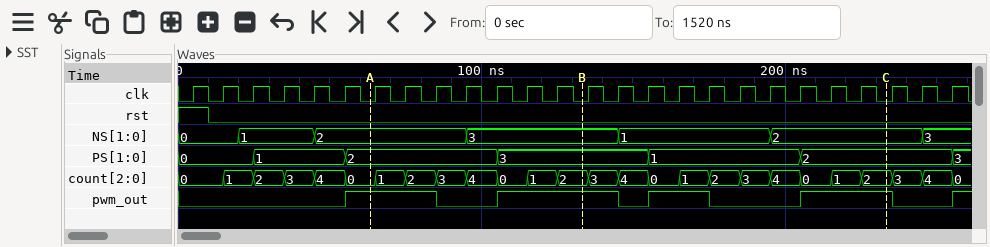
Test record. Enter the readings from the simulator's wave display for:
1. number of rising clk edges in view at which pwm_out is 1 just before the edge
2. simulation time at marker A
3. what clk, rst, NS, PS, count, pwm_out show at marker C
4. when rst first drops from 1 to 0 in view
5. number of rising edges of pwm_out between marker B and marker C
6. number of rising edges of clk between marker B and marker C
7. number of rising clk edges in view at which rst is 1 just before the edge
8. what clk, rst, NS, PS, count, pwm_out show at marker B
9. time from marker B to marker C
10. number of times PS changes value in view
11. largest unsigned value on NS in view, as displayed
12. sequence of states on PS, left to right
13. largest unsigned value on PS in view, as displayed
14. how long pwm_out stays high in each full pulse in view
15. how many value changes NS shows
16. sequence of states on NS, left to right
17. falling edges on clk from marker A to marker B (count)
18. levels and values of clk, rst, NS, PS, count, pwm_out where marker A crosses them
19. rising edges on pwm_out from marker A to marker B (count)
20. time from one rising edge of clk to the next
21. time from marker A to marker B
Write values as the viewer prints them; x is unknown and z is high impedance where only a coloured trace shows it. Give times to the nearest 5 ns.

12
65 ns
clk=0, rst=0, NS=2, PS=2, count=2, pwm_out=1
10 ns
2
10
1
clk=0, rst=0, NS=3, PS=3, count=2, pwm_out=1
100 ns
6
3
0, 1, 2, 3, 1, 2, 3
3
30 ns, 40 ns, 20 ns, 30 ns
6
0, 1, 2, 3, 1, 2, 3
7
clk=0, rst=0, NS=2, PS=2, count=0, pwm_out=1
1
10 ns
70 ns
